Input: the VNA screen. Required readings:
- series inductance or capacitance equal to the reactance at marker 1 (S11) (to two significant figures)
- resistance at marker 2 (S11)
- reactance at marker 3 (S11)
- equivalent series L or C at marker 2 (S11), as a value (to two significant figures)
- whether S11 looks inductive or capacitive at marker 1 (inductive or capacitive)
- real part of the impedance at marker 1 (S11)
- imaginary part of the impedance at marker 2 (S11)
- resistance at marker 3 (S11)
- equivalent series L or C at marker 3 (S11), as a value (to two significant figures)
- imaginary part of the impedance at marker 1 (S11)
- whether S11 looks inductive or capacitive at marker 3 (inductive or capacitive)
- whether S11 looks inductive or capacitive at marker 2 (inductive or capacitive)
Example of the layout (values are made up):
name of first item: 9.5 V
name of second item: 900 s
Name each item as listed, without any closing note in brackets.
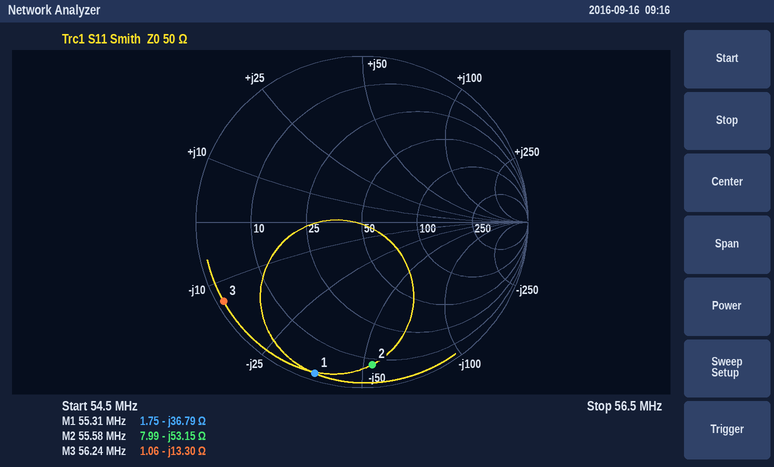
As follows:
series inductance or capacitance equal to the reactance at marker 1 (S11): 78 pF
resistance at marker 2: 7.99 Ω
reactance at marker 3: -13.30 Ω
equivalent series L or C at marker 2 (S11), as a value: 54 pF
whether S11 looks inductive or capacitive at marker 1: capacitive
real part of the impedance at marker 1: 1.75 Ω
imaginary part of the impedance at marker 2: -53.15 Ω
resistance at marker 3: 1.06 Ω
equivalent series L or C at marker 3 (S11), as a value: 210 pF
imaginary part of the impedance at marker 1: -36.79 Ω
whether S11 looks inductive or capacitive at marker 3: capacitive
whether S11 looks inductive or capacitive at marker 2: capacitive
